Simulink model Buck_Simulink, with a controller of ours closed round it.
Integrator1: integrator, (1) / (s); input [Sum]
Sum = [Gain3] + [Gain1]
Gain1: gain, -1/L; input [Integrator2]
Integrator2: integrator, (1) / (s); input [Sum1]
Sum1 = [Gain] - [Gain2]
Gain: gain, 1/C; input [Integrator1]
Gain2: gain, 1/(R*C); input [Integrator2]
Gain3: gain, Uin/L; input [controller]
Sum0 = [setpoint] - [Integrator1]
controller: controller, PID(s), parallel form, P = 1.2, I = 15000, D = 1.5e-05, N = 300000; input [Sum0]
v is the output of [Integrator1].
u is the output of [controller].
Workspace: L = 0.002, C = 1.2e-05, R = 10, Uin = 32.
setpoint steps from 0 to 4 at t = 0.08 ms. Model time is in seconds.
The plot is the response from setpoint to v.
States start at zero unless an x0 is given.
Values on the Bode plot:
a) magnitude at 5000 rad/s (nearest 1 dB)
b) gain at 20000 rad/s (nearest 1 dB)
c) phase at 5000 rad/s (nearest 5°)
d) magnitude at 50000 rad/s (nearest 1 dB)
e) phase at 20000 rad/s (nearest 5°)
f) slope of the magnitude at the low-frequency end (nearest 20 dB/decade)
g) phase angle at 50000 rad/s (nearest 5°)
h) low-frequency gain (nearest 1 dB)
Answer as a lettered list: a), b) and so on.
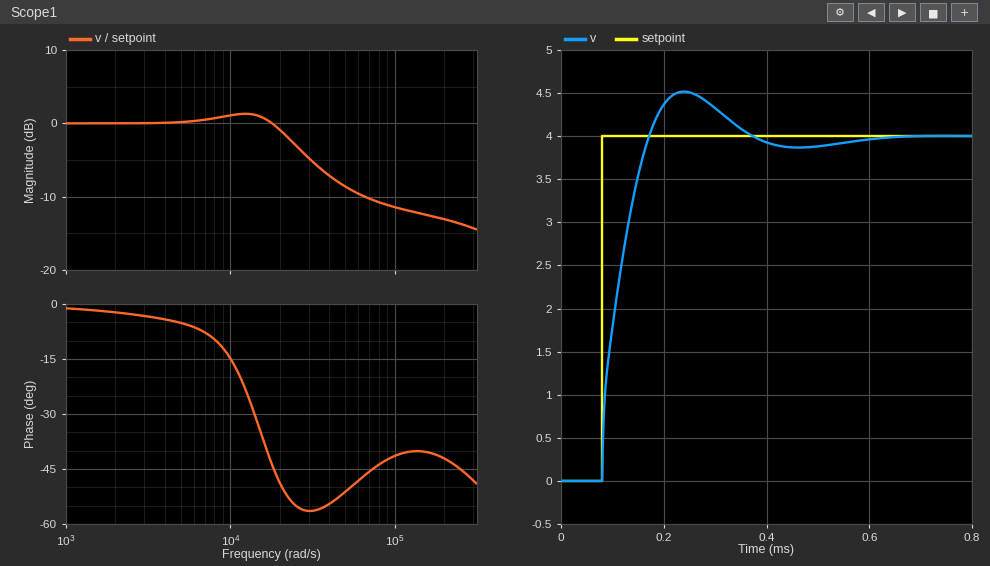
a) 0 dB
b) -1 dB
c) -5°
d) -9 dB
e) -50°
f) 0 dB/decade
g) -50°
h) 0 dB
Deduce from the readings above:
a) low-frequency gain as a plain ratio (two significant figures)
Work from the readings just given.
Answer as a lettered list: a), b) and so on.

a) 1.0
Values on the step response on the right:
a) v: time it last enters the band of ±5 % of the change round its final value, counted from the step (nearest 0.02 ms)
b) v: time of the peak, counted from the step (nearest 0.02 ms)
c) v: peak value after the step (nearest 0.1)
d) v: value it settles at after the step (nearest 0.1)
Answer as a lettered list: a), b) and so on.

a) 0.24 ms
b) 0.16 ms
c) 4.5
d) 4.0
